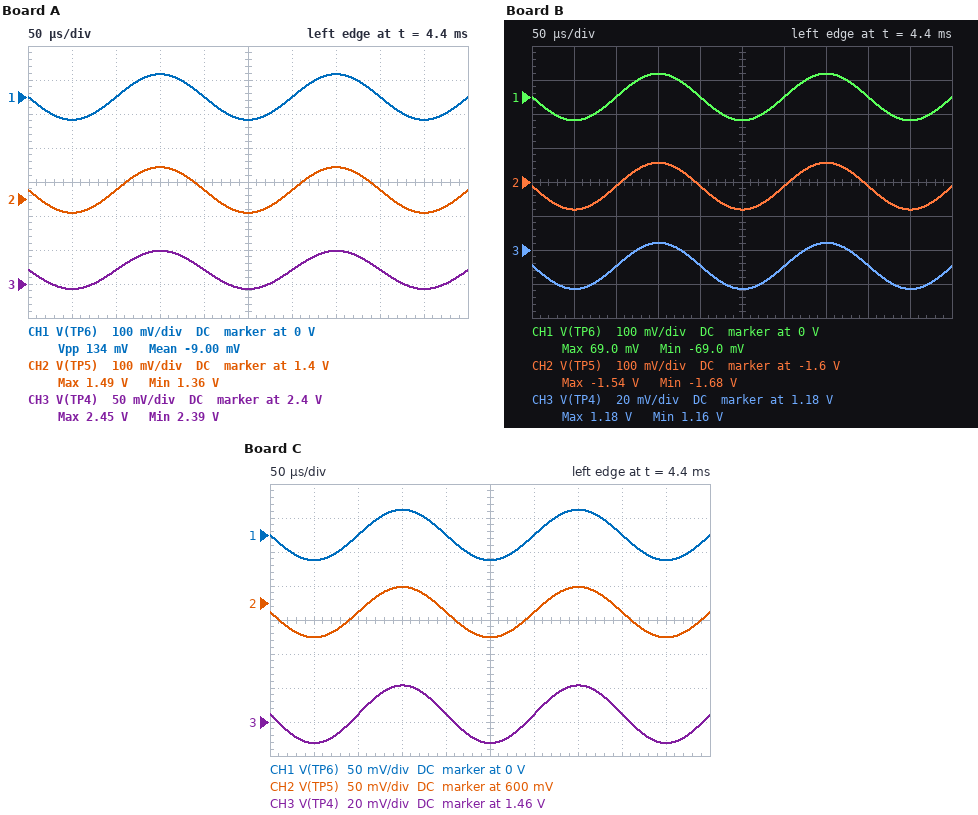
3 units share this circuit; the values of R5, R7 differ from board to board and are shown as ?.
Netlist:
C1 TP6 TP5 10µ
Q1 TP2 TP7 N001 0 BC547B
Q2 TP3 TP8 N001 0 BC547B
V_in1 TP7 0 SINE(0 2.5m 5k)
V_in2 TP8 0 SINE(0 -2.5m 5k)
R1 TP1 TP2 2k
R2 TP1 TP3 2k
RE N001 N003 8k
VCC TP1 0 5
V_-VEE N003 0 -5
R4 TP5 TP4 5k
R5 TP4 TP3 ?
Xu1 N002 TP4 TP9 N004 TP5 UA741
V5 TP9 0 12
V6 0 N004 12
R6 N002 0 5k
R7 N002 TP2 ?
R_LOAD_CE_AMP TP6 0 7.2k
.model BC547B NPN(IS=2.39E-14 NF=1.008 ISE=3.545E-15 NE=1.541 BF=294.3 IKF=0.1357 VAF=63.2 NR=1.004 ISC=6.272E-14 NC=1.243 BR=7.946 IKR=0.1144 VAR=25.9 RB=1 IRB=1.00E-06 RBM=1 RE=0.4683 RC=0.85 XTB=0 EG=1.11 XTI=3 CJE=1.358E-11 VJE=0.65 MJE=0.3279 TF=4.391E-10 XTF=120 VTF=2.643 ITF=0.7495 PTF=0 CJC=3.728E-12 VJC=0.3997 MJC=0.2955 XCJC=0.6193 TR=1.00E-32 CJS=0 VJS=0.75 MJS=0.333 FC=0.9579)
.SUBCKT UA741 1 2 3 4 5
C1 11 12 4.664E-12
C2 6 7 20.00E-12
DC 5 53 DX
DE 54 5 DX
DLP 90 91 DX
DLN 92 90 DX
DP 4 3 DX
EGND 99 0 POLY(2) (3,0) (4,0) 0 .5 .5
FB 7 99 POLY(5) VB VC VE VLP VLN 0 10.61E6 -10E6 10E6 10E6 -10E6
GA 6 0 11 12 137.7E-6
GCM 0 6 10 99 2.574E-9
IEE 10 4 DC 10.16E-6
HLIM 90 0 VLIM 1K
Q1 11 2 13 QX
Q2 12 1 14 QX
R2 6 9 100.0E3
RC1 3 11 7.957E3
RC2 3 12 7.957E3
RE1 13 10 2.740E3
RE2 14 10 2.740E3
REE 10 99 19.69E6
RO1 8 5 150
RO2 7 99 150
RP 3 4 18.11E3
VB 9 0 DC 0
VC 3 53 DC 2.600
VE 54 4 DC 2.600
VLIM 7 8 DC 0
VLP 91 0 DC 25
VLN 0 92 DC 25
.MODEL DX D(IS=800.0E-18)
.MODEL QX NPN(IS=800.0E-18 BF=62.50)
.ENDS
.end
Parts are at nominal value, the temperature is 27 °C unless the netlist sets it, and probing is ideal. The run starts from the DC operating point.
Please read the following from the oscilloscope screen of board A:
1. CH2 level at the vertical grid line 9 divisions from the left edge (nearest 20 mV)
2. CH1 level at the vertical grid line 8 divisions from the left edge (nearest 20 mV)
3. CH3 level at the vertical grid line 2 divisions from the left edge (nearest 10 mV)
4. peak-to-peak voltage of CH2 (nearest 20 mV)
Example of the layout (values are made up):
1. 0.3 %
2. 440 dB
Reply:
1. 1.36 V
2. 0 V
3. 2.42 V
4. 140 mV
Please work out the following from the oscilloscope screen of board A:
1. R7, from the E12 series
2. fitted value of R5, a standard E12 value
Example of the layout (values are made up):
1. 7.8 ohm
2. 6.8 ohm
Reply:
1. 2.2 kΩ
2. 8.2 kΩ
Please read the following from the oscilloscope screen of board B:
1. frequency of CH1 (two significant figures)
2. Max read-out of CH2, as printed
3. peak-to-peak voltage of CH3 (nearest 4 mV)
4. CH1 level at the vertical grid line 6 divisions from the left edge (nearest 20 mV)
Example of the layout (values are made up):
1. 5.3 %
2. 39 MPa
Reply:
1. 5.0 kHz
2. -1.54 V
3. 28 mV
4. 0 V
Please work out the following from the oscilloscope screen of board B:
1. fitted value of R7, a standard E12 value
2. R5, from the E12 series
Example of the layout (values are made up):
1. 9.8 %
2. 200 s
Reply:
1. 12 kΩ
2. 3.9 kΩ
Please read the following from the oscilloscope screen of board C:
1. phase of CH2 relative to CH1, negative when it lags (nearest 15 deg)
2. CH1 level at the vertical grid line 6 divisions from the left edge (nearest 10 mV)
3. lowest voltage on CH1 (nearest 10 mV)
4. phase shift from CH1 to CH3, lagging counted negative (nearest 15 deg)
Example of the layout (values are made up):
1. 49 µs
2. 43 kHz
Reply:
1. 0 deg
2. 0 V
3. -40 mV
4. 0 deg
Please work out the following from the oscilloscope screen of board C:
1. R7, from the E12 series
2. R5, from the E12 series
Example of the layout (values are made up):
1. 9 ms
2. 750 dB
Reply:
1. 8.2 kΩ
2. 15 kΩ
